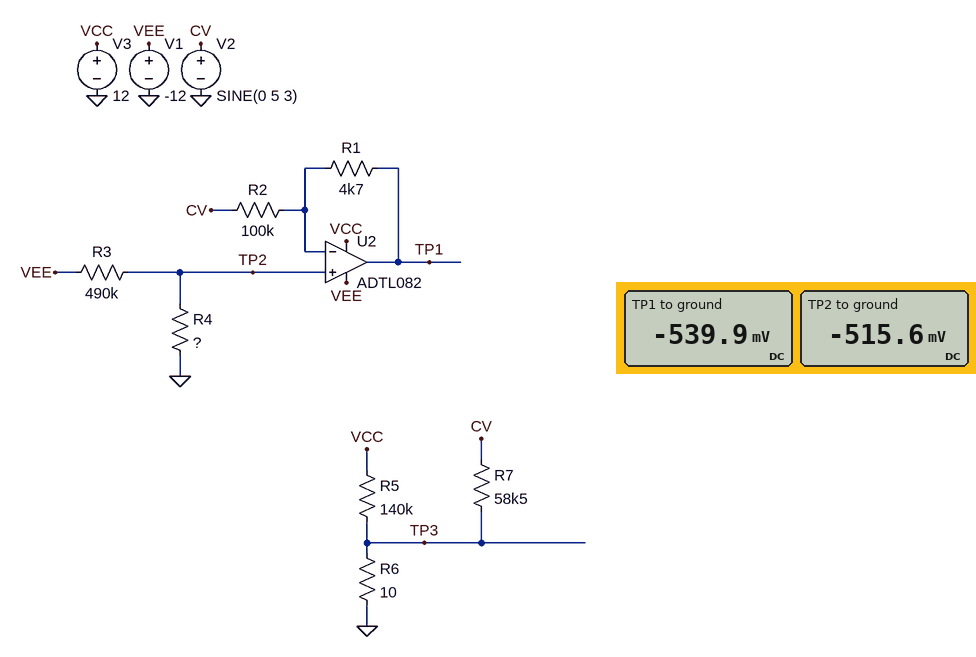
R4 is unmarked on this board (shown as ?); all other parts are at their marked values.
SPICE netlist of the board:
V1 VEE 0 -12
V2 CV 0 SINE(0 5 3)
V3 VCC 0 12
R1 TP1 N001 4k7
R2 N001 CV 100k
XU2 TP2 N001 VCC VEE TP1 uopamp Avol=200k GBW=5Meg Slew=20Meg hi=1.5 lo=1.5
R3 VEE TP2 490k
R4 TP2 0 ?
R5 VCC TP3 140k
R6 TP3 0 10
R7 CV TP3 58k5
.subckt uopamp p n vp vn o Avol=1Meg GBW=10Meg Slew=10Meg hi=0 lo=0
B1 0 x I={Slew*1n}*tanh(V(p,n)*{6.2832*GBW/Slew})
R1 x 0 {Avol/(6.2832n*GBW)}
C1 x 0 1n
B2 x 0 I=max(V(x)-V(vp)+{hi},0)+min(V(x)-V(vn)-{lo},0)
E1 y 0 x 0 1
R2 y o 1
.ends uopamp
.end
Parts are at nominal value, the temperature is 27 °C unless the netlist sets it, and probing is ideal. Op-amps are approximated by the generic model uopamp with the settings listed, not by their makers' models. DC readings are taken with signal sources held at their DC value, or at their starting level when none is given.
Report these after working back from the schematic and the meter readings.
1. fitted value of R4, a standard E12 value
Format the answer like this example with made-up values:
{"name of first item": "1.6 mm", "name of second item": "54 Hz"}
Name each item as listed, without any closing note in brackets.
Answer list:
{"fitted value of R4, a standard E12 value": "22 kΩ"}
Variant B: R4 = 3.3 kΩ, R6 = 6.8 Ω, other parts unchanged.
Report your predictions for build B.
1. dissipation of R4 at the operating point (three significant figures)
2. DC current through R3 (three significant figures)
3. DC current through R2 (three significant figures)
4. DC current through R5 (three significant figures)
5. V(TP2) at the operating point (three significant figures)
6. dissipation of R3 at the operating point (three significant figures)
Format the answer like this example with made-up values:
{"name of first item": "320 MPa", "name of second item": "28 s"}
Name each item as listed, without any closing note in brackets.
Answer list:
{"dissipation of R4 at the operating point": "1.95 µW", "DC current through R3": "24.3 µA", "DC current through R2": "803 nA", "DC current through R5": "85.7 µA", "V(TP2) at the operating point": "-80.3 mV", "dissipation of R3 at the operating point": "290 µW"}
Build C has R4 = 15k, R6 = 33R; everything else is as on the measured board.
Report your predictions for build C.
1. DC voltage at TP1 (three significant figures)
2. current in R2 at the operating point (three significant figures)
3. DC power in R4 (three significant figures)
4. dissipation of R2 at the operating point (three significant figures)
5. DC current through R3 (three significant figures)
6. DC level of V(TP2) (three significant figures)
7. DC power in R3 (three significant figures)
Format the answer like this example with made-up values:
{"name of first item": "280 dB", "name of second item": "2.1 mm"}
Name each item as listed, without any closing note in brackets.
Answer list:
{"DC voltage at TP1": "-373 mV", "current in R2 at the operating point": "3.56 µA", "DC power in R4": "8.47 µW", "dissipation of R2 at the operating point": "1.27 µW", "DC current through R3": "23.8 µA", "DC level of V(TP2)": "-356 mV", "DC power in R3": "277 µW"}
